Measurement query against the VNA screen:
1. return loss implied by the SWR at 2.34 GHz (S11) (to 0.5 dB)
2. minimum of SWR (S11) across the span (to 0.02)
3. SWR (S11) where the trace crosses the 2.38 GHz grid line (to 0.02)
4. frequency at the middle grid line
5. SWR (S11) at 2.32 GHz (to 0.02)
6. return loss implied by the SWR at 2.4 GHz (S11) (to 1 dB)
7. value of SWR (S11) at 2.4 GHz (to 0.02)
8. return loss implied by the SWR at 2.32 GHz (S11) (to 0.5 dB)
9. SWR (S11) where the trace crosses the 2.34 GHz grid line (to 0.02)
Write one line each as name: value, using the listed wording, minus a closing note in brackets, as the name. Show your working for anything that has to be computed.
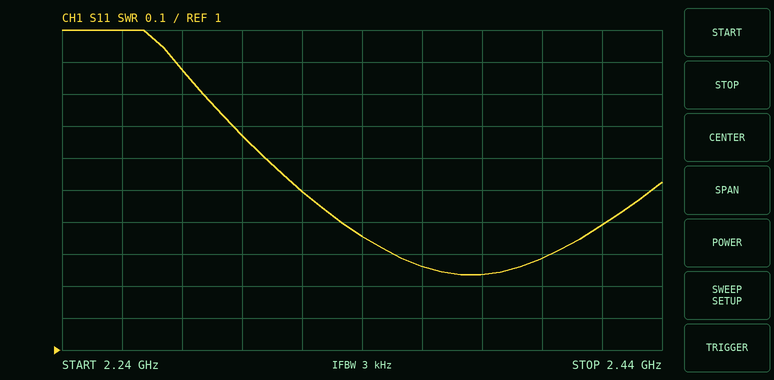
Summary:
return loss implied by the SWR at 2.34 GHz (S11): −20 log10((1.36 − 1)/(1.36 + 1)) ≈ 16.3 dB, so 16.5 dB to the nearest 0.5 dB
minimum of SWR (S11) across the span: 1.24
SWR (S11) where the trace crosses the 2.38 GHz grid line: 1.24
frequency at the middle grid line: 2.34 GHz
SWR (S11) at 2.32 GHz: 1.50
return loss implied by the SWR at 2.4 GHz (S11): −20 log10((1.28 − 1)/(1.28 + 1)) ≈ 18 dB
value of SWR (S11) at 2.4 GHz: 1.28
return loss implied by the SWR at 2.32 GHz (S11): −20 log10((1.5 − 1)/(1.5 + 1)) ≈ 14.0 dB
SWR (S11) where the trace crosses the 2.34 GHz grid line: 1.36
